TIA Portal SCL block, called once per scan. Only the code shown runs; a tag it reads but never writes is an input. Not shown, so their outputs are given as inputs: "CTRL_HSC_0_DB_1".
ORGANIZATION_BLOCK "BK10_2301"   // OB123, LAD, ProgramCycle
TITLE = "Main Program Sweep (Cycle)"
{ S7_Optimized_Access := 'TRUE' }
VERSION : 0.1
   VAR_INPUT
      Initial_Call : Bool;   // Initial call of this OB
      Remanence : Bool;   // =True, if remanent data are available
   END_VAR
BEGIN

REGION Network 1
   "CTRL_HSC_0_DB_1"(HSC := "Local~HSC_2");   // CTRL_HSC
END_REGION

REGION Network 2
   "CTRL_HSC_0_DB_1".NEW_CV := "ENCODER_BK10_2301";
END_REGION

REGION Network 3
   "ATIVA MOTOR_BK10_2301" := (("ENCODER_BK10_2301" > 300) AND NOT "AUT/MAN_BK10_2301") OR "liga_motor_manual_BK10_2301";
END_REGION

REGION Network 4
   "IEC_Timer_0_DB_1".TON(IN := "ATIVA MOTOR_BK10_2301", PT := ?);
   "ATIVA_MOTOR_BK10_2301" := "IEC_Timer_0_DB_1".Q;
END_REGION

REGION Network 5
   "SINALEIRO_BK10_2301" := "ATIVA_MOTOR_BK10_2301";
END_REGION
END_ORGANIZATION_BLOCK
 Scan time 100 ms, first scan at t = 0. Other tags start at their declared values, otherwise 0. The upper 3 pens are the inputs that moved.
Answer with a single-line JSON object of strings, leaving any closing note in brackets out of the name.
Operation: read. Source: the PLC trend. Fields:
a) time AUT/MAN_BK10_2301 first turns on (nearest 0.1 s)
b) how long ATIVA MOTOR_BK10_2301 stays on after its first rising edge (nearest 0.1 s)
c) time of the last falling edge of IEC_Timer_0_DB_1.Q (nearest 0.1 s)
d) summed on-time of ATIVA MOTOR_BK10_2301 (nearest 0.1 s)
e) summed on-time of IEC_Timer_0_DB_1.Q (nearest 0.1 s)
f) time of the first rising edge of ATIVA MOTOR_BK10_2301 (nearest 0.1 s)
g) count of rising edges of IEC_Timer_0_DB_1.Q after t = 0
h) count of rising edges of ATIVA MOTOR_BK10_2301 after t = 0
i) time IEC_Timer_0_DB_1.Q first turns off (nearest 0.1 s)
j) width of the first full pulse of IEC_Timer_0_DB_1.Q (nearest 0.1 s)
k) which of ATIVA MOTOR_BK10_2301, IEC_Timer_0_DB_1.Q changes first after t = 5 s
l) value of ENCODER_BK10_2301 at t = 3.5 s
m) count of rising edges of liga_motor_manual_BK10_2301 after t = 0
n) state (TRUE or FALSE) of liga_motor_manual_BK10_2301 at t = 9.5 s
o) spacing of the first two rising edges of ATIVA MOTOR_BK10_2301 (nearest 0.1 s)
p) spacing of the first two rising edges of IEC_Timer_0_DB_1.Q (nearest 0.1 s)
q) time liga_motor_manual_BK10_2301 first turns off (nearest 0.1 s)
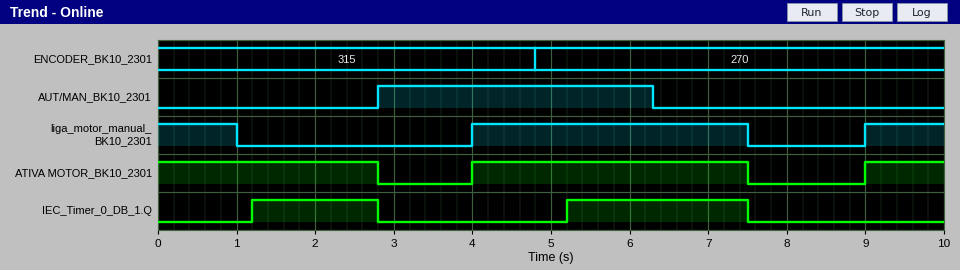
{"time AUT/MAN_BK10_2301 first turns on": "2.8 s", "how long ATIVA MOTOR_BK10_2301 stays on after its first rising edge": "3.5 s", "time of the last falling edge of IEC_Timer_0_DB_1.Q": "7.5 s", "summed on-time of ATIVA MOTOR_BK10_2301": "7.3 s", "summed on-time of IEC_Timer_0_DB_1.Q": "3.9 s", "time of the first rising edge of ATIVA MOTOR_BK10_2301": "4.0 s", "count of rising edges of IEC_Timer_0_DB_1.Q after t = 0": "2", "count of rising edges of ATIVA MOTOR_BK10_2301 after t = 0": "2", "time IEC_Timer_0_DB_1.Q first turns off": "2.8 s", "width of the first full pulse of IEC_Timer_0_DB_1.Q": "1.6 s", "which of ATIVA MOTOR_BK10_2301, IEC_Timer_0_DB_1.Q changes first after t = 5 s": "IEC_Timer_0_DB_1.Q", "value of ENCODER_BK10_2301 at t = 3.5 s": "315", "count of rising edges of liga_motor_manual_BK10_2301 after t = 0": "2", "state (TRUE or FALSE) of liga_motor_manual_BK10_2301 at t = 9.5 s": "TRUE", "spacing of the first two rising edges of ATIVA MOTOR_BK10_2301": "5.0 s", "spacing of the first two rising edges of IEC_Timer_0_DB_1.Q": "4.0 s", "time liga_motor_manual_BK10_2301 first turns off": "1.0 s"}
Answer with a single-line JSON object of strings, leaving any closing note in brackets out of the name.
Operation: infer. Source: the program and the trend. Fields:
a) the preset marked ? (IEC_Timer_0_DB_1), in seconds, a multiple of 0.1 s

{"the preset marked ? (IEC_Timer_0_DB_1), in seconds, a multiple of 0.1 s": "1.2 s"}
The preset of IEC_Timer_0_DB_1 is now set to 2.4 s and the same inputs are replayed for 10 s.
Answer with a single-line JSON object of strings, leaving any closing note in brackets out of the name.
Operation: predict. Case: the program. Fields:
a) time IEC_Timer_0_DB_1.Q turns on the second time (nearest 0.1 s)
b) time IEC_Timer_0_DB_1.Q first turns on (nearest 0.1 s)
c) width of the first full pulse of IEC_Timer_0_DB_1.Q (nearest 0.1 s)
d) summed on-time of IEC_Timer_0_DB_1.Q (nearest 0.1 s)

{"time IEC_Timer_0_DB_1.Q turns on the second time": "6.4 s", "time IEC_Timer_0_DB_1.Q first turns on": "2.4 s", "width of the first full pulse of IEC_Timer_0_DB_1.Q": "0.4 s", "summed on-time of IEC_Timer_0_DB_1.Q": "1.5 s"}
